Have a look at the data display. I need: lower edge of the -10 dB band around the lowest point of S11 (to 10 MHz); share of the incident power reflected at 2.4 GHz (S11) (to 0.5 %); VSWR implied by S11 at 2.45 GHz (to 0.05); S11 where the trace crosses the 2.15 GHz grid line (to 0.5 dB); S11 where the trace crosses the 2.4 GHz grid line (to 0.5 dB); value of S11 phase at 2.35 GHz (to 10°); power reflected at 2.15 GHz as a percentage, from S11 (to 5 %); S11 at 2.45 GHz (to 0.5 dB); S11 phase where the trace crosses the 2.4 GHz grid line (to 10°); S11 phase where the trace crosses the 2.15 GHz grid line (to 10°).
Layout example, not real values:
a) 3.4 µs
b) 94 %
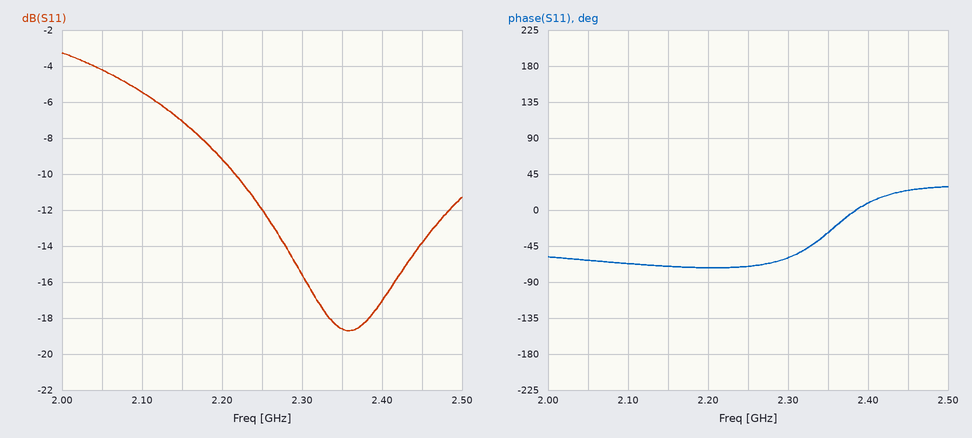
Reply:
a) 2.22 GHz
b) 2.0 %
c) 1.50
d) -7.0 dB
e) -17.0 dB
f) -30°
g) 20 %
h) -14.0 dB
i) 10°
j) -70°
